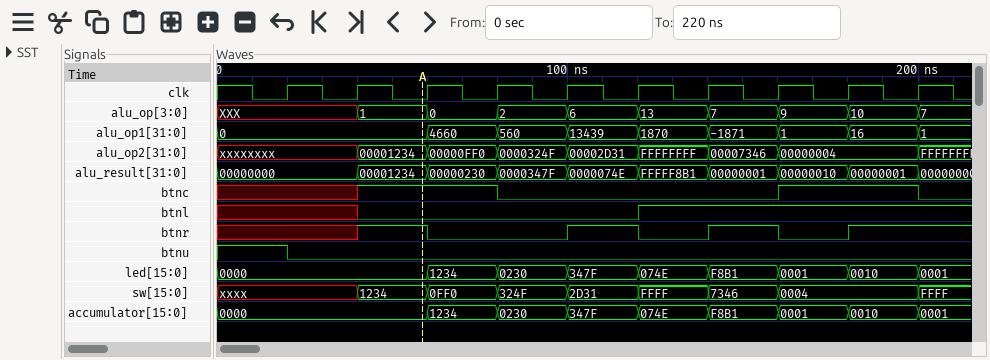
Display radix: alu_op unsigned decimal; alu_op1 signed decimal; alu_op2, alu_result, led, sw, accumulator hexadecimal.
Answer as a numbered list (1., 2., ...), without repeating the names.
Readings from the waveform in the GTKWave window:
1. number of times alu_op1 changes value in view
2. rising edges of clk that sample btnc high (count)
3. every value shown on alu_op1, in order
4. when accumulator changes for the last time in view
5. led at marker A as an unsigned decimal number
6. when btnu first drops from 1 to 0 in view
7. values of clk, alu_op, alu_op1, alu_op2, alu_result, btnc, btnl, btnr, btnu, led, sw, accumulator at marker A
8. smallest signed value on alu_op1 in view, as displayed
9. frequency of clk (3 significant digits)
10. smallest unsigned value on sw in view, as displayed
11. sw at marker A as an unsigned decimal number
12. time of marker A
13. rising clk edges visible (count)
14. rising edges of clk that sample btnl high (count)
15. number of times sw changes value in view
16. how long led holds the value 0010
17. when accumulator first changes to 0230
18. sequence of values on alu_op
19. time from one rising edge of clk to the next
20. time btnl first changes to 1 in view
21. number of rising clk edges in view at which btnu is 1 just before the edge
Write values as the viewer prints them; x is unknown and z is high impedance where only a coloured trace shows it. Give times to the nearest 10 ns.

1. 8
2. 4
3. 0, 4660, 560, 13439, 1870, -1871, 1, 16, 1
4. 200 ns
5. 0
6. 20 ns
7. clk=0, alu_op=1, alu_op1=0, alu_op2=00001234, alu_result=00001234, btnc=1, btnl=0, btnr=1, btnu=0, led=0000, sw=1234, accumulator=0000
8. -1871
9. 50.0 MHz
10. 0004
11. 4660
12. 60 ns
13. 10
14. 4
15. 8
16. 20 ns
17. 80 ns
18. XXX, 1, 0, 2, 6, 13, 7, 9, 10, 7
19. 20 ns
20. 120 ns
21. 1
